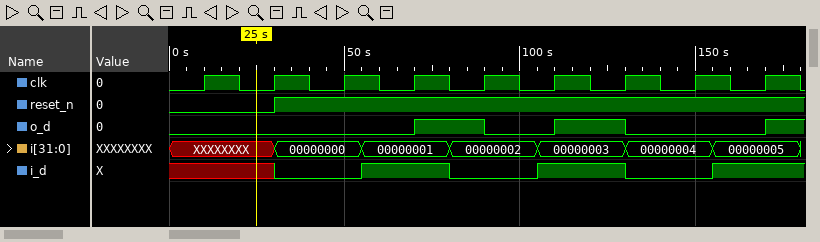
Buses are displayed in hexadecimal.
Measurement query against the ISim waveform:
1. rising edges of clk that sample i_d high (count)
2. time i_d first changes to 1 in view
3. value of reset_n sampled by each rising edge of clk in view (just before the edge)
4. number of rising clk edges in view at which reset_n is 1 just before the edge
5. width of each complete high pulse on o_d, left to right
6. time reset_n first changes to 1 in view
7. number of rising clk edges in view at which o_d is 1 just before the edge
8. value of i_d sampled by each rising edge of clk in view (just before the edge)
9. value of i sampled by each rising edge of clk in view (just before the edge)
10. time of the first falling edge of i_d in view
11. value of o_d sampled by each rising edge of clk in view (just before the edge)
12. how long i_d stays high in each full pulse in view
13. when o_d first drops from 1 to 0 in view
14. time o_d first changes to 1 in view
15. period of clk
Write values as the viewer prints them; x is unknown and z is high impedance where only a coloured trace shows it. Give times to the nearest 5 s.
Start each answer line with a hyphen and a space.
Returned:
- 4
- 55 s
- 0 0 1 1 1 1 1 1 1
- 7
- 20 s, 20 s
- 30 s
- 2
- x x 0 1 0 1 1 0 1
- XXXXXXXX, XXXXXXXX, 00000000, 00000001, 00000002, 00000003, 00000003, 00000004, 00000005
- 80 s
- 0 0 0 0 1 0 1 0 0
- 25 s, 25 s
- 90 s
- 70 s
- 20 s
